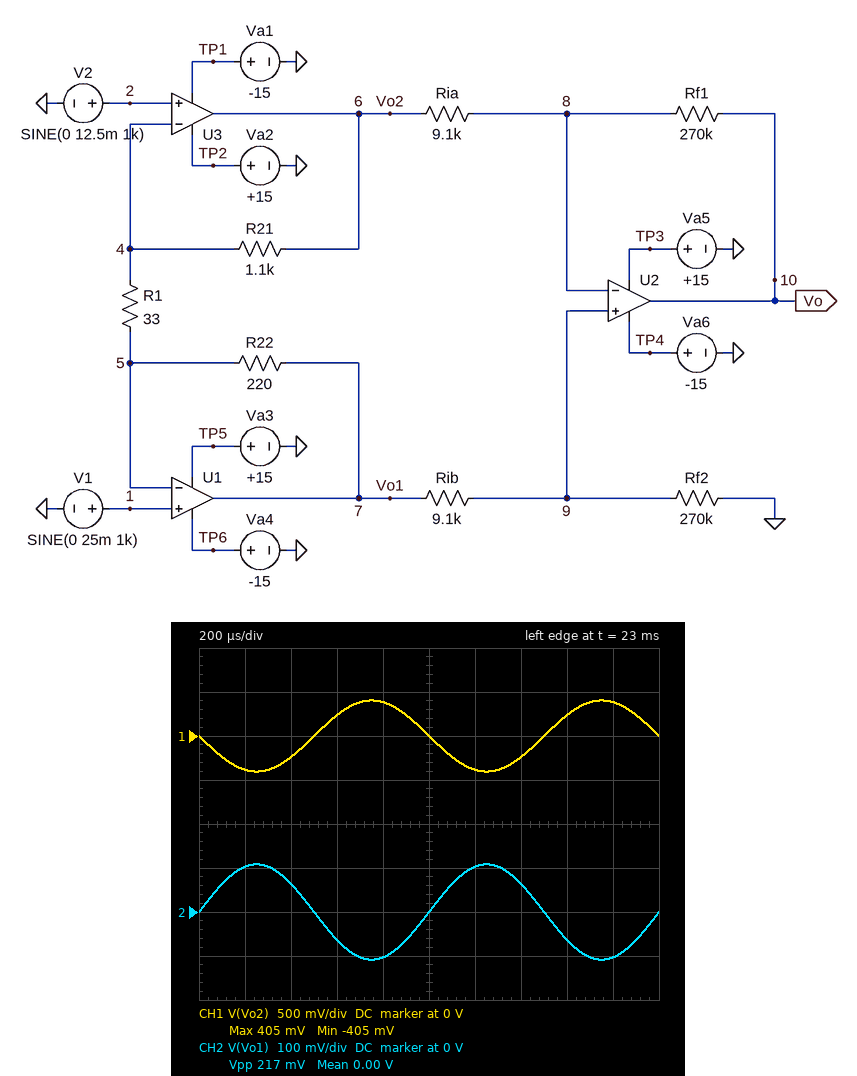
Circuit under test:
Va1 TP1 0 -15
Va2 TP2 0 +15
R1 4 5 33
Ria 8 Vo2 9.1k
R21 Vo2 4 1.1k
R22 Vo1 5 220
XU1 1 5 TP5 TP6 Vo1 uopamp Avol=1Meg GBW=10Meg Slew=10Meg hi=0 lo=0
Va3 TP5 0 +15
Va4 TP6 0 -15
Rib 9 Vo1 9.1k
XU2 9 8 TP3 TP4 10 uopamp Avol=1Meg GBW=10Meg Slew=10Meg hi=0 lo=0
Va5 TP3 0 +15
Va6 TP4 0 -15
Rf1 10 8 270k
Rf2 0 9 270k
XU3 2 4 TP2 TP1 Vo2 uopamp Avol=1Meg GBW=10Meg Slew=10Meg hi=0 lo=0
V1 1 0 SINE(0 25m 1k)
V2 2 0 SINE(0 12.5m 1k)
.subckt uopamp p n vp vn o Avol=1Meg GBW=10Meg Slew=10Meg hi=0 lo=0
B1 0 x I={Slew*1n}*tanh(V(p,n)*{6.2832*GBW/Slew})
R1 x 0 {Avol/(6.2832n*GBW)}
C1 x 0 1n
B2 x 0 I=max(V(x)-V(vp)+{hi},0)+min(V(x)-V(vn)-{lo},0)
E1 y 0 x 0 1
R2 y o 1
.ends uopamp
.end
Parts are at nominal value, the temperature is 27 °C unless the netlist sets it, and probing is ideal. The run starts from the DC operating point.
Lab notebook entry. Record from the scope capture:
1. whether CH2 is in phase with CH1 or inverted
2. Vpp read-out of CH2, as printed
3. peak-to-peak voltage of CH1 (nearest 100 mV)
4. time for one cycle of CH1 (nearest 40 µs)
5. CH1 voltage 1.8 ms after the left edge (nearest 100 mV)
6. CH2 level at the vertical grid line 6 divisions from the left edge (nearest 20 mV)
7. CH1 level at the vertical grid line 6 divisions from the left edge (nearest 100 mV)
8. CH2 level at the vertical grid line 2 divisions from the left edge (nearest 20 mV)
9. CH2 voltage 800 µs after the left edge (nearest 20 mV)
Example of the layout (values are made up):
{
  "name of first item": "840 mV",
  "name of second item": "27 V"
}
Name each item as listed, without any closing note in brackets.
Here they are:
{
  "whether CH2 is in phase with CH1 or inverted": "inverted",
  "Vpp read-out of CH2, as printed": "217 mV",
  "peak-to-peak voltage of CH1": "800 mV",
  "time for one cycle of CH1": "1.00 ms",
  "CH1 voltage 1.8 ms after the left edge": "400 mV",
  "CH2 level at the vertical grid line 6 divisions from the left edge": "100 mV",
  "CH1 level at the vertical grid line 6 divisions from the left edge": "-400 mV",
  "CH2 level at the vertical grid line 2 divisions from the left edge": "60 mV",
  "CH2 voltage 800 µs after the left edge": "-100 mV"
}
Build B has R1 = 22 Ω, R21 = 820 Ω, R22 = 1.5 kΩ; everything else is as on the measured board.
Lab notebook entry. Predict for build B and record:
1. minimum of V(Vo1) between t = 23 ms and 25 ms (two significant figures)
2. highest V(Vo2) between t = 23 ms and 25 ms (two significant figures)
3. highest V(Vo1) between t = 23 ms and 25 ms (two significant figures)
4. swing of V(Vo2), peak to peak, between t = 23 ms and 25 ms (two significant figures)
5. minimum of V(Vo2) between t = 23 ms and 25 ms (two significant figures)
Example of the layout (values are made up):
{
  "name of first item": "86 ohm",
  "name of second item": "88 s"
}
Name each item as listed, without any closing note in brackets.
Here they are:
{
  "minimum of V(Vo1) between t = 23 ms and 25 ms": "-880 mV",
  "highest V(Vo2) between t = 23 ms and 25 ms": "450 mV",
  "highest V(Vo1) between t = 23 ms and 25 ms": "880 mV",
  "swing of V(Vo2), peak to peak, between t = 23 ms and 25 ms": "910 mV",
  "minimum of V(Vo2) between t = 23 ms and 25 ms": "-450 mV"
}
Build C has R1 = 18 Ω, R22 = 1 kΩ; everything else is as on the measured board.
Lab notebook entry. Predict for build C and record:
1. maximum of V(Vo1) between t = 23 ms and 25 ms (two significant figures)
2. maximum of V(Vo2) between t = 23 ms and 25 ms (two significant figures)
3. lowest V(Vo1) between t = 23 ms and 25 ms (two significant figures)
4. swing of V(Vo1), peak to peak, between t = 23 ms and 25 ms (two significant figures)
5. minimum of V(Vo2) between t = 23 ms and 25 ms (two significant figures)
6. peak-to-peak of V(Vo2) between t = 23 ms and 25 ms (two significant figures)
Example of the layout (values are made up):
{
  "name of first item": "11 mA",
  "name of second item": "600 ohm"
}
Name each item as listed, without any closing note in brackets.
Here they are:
{
  "maximum of V(Vo1) between t = 23 ms and 25 ms": "720 mV",
  "maximum of V(Vo2) between t = 23 ms and 25 ms": "750 mV",
  "lowest V(Vo1) between t = 23 ms and 25 ms": "-720 mV",
  "swing of V(Vo1), peak to peak, between t = 23 ms and 25 ms": "1.4 V",
  "minimum of V(Vo2) between t = 23 ms and 25 ms": "-750 mV",
  "peak-to-peak of V(Vo2) between t = 23 ms and 25 ms": "1.5 V"
}
